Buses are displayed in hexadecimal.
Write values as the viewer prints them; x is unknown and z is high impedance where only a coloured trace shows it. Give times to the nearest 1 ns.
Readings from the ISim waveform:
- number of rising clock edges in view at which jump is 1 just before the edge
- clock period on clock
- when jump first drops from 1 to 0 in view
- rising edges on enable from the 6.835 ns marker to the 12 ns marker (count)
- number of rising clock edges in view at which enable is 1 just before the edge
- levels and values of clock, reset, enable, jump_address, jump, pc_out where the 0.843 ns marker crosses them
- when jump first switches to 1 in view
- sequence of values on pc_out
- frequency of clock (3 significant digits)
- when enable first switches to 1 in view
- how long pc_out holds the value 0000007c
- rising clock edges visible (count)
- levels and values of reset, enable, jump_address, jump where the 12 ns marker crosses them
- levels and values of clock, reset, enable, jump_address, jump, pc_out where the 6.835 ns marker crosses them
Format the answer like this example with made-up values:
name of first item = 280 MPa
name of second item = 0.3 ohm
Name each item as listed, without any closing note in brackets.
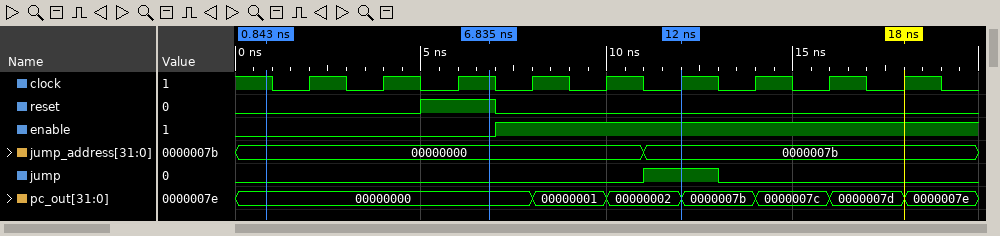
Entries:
number of rising clock edges in view at which jump is 1 just before the edge = 1
clock period on clock = 2 ns
when jump first drops from 1 to 0 in view = 13 ns
rising edges on enable from the 6.835 ns marker to the 12 ns marker = 1
number of rising clock edges in view at which enable is 1 just before the edge = 6
levels and values of clock, reset, enable, jump_address, jump, pc_out where the 0.843 ns marker crosses them = clock=1, reset=0, enable=0, jump_address=00000000, jump=0, pc_out=00000000
when jump first switches to 1 in view = 11 ns
sequence of values on pc_out = 00000000, 00000001, 00000002, 0000007b, 0000007c, 0000007d, 0000007e
frequency of clock = 500 MHz
when enable first switches to 1 in view = 7 ns
how long pc_out holds the value 0000007c = 2 ns
rising clock edges visible = 9
levels and values of reset, enable, jump_address, jump where the 12 ns marker crosses them = reset=0, enable=1, jump_address=0000007b, jump=1
levels and values of clock, reset, enable, jump_address, jump, pc_out where the 6.835 ns marker crosses them = clock=1, reset=1, enable=0, jump_address=00000000, jump=0, pc_out=00000000
